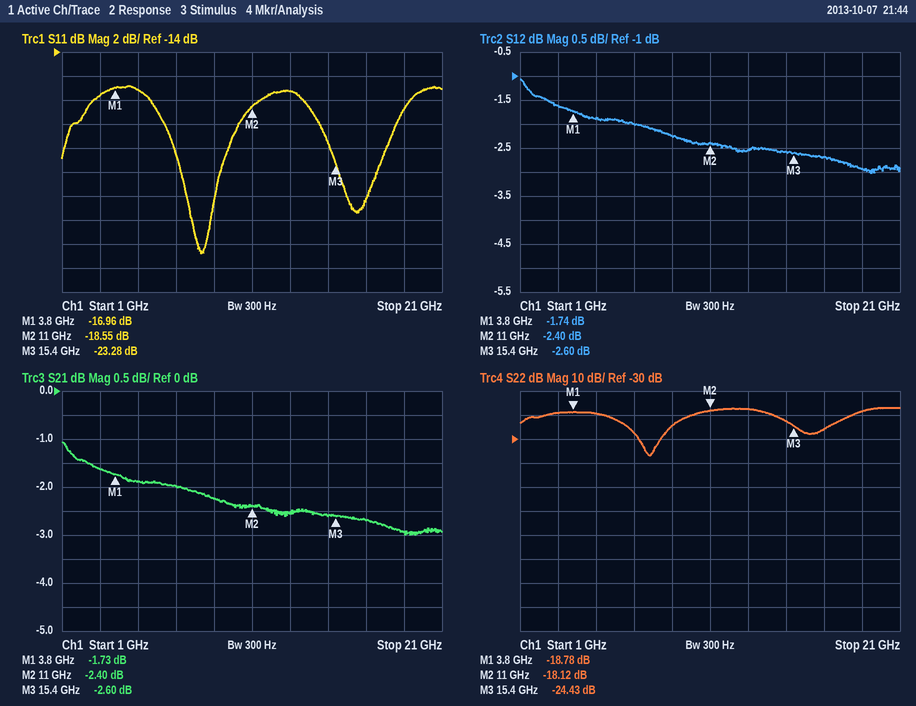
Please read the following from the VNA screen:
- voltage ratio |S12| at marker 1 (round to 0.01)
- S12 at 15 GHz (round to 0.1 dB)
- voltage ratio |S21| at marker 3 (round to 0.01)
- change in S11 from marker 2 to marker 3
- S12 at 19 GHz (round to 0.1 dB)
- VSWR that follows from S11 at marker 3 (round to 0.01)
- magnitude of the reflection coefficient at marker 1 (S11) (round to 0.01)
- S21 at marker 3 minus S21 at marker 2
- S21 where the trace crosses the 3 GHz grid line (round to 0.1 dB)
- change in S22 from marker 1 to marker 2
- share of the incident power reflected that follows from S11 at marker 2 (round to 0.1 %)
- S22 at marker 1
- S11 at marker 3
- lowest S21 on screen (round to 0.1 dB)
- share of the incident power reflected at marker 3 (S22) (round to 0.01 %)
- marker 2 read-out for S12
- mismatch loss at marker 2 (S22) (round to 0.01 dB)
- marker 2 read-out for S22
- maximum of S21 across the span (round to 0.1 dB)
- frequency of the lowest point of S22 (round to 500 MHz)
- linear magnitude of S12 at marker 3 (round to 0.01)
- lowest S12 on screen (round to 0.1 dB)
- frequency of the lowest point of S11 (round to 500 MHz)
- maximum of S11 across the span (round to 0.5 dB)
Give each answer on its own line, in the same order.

0.82
-2.6 dB
0.74
-4.73 dB
-2.9 dB
1.15
0.14
-0.20 dB
-1.6 dB
0.66 dB
1.4 %
-18.78 dB
-23.28 dB
-3.0 dB
0.36 %
-2.40 dB
0.07 dB
-18.12 dB
-1.1 dB
8.0 GHz
0.74
-3.0 dB
8.5 GHz
-17.0 dB
